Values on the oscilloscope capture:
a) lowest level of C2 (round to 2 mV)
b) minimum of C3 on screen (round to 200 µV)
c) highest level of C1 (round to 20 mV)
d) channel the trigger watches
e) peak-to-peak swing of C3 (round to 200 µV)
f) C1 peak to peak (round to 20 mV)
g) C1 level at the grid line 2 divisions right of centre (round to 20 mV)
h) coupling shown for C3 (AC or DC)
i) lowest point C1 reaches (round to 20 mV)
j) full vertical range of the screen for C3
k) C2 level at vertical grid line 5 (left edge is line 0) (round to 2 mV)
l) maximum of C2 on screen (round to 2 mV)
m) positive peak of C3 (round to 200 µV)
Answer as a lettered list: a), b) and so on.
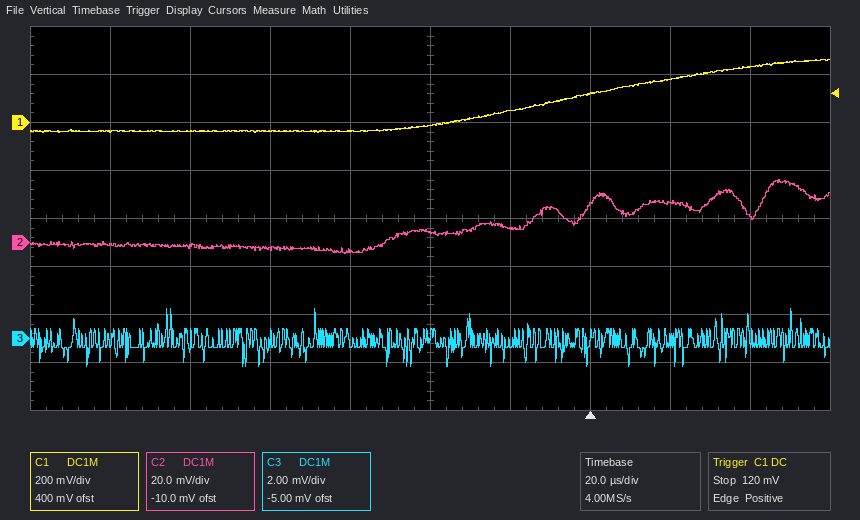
a) -4 mV
b) -1.2 mV
c) 260 mV
d) C1
e) 2.4 mV
f) 300 mV
g) 120 mV
h) DC
i) -40 mV
j) 16 mV
k) 4 mV
l) 26 mV
m) 1.2 mV
